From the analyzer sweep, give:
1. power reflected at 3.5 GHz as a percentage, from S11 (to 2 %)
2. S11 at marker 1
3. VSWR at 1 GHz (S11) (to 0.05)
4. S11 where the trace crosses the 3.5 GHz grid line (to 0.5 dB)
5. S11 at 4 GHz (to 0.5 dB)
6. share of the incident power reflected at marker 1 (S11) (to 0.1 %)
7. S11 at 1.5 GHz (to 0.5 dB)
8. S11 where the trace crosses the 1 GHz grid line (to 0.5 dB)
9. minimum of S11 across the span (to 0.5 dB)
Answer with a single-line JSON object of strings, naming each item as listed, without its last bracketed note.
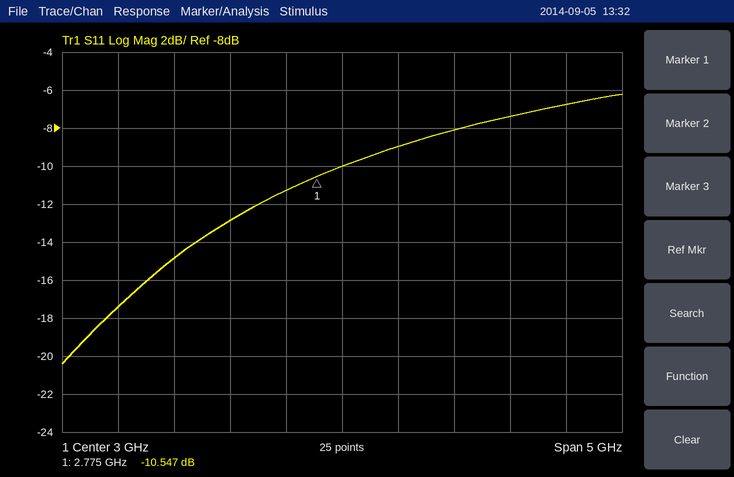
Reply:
{"power reflected at 3.5 GHz as a percentage, from S11": "12 %", "S11 at marker 1": "-10.547 dB", "VSWR at 1 GHz (S11)": "1.30", "S11 where the trace crosses the 3.5 GHz grid line": "-9.0 dB", "S11 at 4 GHz": "-8.0 dB", "share of the incident power reflected at marker 1 (S11)": "8.8 %", "S11 at 1.5 GHz": "-15.0 dB", "S11 where the trace crosses the 1 GHz grid line": "-17.5 dB", "minimum of S11 across the span": "-20.5 dB"}
